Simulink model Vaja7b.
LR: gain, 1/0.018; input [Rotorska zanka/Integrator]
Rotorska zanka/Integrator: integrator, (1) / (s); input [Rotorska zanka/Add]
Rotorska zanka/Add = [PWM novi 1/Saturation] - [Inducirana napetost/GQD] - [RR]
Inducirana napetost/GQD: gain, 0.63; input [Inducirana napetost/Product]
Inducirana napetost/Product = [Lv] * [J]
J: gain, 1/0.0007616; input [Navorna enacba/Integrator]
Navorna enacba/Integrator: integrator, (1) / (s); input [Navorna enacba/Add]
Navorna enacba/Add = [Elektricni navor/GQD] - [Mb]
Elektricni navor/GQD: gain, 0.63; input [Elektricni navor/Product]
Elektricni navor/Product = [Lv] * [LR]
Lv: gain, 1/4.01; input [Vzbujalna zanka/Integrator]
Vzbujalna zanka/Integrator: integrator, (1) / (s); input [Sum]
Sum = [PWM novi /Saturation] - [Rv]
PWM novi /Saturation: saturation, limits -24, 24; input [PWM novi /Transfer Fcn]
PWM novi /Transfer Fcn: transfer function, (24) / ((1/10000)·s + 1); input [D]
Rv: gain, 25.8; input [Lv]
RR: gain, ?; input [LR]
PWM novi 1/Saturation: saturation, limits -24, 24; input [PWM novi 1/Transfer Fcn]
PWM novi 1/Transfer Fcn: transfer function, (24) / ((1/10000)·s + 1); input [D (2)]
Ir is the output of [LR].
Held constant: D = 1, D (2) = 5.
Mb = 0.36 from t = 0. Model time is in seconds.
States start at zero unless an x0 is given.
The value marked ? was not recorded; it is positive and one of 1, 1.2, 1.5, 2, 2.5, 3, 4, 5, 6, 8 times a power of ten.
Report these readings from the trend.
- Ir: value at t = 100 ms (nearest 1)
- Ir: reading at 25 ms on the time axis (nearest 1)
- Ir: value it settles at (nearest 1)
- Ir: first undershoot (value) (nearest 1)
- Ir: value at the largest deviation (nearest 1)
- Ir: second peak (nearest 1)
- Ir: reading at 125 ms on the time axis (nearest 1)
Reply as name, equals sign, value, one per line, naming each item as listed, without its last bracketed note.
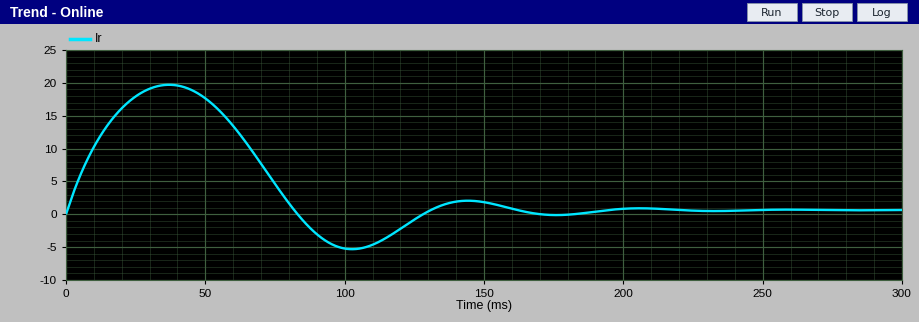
Ir: value at t = 100 ms = -5
Ir: reading at 25 ms on the time axis = 18
Ir: value it settles at = 1
Ir: first undershoot (value) = -5
Ir: value at the largest deviation = 20
Ir: second peak = 2
Ir: reading at 125 ms on the time axis = -1
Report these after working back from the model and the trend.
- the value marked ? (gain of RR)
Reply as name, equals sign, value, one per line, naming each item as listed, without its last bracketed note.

the value marked ? = 1
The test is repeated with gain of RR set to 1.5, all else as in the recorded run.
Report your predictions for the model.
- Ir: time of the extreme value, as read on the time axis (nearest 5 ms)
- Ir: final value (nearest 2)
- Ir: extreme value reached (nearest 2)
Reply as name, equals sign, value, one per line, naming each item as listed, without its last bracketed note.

Ir: time of the extreme value, as read on the time axis = 35 ms
Ir: final value = 0
Ir: extreme value reached = 14
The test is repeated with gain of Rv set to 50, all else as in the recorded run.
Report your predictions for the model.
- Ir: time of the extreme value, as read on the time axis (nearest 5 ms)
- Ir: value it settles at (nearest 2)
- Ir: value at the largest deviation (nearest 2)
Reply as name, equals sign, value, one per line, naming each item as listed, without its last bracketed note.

Ir: time of the extreme value, as read on the time axis = 40 ms
Ir: value it settles at = 2
Ir: value at the largest deviation = 20
